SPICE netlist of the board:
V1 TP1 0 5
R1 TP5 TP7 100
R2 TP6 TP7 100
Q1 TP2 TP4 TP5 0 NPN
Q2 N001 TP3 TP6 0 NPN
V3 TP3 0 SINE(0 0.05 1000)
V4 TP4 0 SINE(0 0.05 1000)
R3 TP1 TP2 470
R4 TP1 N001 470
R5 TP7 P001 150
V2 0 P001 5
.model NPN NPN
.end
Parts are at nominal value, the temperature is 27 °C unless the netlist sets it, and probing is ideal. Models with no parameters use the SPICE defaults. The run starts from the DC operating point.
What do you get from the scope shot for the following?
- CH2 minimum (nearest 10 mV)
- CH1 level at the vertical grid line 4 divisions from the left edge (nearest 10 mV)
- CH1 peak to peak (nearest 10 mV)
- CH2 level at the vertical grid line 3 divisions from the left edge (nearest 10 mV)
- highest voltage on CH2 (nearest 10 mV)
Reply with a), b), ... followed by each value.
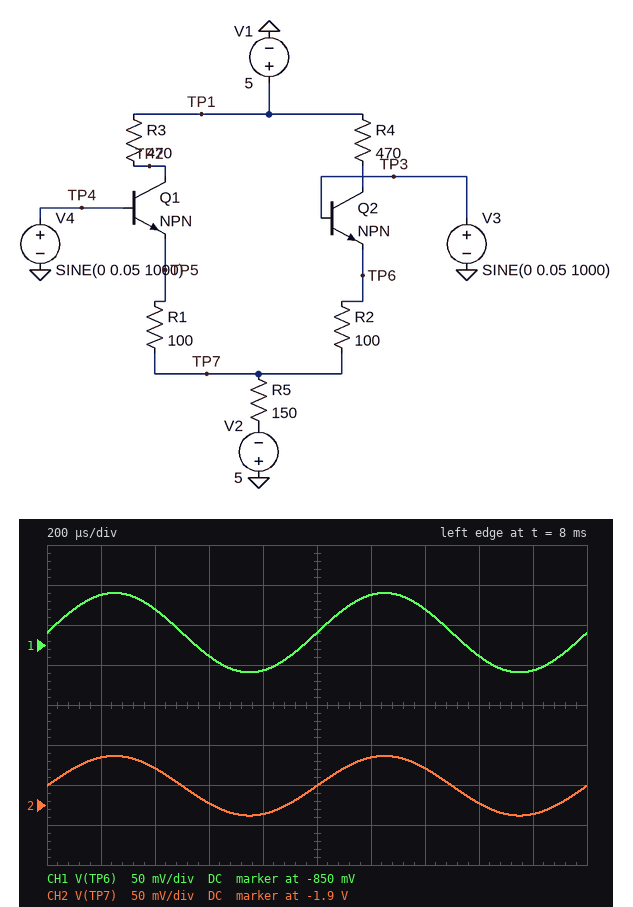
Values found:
a) -1.91 V
b) -880 mV
c) 100 mV
d) -1.90 V
e) -1.84 V
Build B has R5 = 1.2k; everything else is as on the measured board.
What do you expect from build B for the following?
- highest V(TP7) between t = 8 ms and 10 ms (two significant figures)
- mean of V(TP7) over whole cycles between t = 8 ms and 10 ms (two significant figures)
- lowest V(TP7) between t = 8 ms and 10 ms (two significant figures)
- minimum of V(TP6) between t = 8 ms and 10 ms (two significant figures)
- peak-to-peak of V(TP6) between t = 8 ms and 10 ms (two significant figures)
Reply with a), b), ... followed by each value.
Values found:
a) -910 mV
b) -960 mV
c) -1.0 V
d) -840 mV
e) 99 mV
